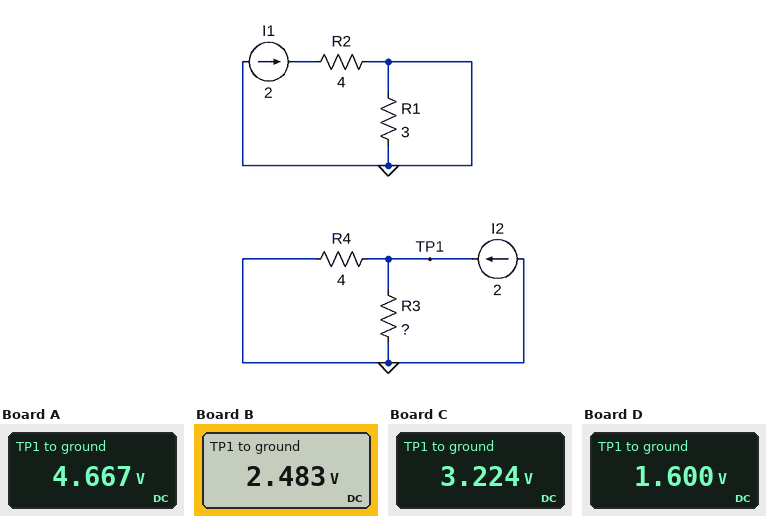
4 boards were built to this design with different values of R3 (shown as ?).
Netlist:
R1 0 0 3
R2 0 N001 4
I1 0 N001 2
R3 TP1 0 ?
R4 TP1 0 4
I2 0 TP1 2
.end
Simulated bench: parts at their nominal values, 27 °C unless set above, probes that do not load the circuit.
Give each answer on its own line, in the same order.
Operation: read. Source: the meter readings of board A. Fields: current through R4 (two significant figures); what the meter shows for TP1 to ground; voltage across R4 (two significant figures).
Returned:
1.2 A
4.667 V
4.7 V
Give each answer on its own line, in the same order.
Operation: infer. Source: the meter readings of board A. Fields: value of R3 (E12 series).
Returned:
5.6 Ω
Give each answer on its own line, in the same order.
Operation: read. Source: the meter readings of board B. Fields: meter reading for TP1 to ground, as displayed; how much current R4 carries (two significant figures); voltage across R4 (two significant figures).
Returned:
2.483 V
620 mA
2.5 V
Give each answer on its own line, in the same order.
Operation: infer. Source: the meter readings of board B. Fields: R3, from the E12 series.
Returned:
1.8 Ω
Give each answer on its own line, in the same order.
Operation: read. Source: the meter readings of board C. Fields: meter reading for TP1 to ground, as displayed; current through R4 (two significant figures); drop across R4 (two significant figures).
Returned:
3.224 V
810 mA
3.2 V
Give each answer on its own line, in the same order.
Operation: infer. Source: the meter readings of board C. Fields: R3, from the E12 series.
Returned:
2.7 Ω
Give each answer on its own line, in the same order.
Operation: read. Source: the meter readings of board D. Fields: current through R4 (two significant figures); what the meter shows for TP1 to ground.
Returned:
400 mA
1.600 V
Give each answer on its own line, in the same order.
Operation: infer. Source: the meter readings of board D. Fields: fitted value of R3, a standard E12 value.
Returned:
1 Ω
